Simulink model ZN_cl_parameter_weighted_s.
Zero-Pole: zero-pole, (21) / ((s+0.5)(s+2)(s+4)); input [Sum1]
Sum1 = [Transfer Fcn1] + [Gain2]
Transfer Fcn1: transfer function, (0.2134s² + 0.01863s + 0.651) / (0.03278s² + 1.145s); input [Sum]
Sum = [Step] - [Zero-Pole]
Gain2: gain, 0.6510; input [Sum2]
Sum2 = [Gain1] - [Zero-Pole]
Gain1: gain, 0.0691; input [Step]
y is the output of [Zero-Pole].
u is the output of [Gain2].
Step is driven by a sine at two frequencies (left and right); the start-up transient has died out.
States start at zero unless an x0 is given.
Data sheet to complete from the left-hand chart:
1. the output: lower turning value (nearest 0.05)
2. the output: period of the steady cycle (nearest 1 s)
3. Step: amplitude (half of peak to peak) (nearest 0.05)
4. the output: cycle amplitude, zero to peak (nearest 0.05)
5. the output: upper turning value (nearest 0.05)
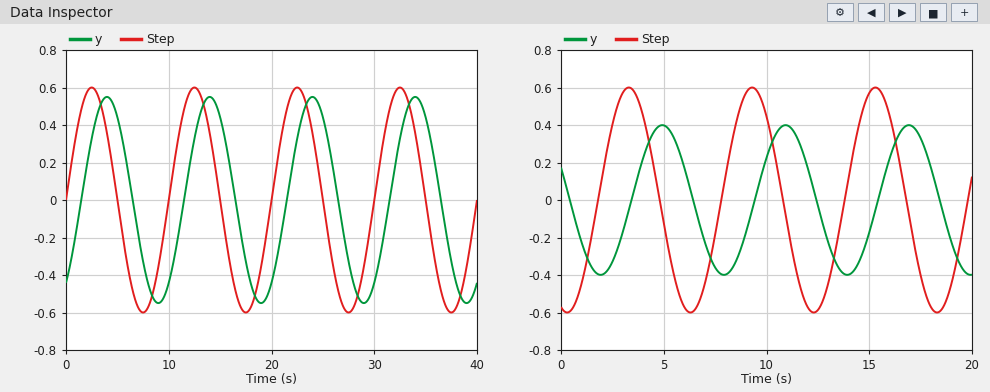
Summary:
-0.55
10 s
0.60
0.55
0.55
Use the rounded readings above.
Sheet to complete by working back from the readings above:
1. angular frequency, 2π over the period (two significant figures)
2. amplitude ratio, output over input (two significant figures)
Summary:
0.63 rad/s
0.92
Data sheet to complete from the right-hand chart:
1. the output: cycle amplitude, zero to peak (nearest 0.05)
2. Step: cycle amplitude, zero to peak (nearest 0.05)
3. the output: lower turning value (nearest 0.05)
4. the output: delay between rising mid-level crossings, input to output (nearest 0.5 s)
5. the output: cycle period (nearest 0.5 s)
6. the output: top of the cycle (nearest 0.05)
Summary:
0.40
0.60
-0.40
1.5 s
6.0 s
0.40
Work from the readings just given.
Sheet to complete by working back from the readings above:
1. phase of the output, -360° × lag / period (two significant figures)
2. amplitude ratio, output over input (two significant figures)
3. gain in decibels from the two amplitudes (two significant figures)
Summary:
-90°
0.67
-3.5 dB
